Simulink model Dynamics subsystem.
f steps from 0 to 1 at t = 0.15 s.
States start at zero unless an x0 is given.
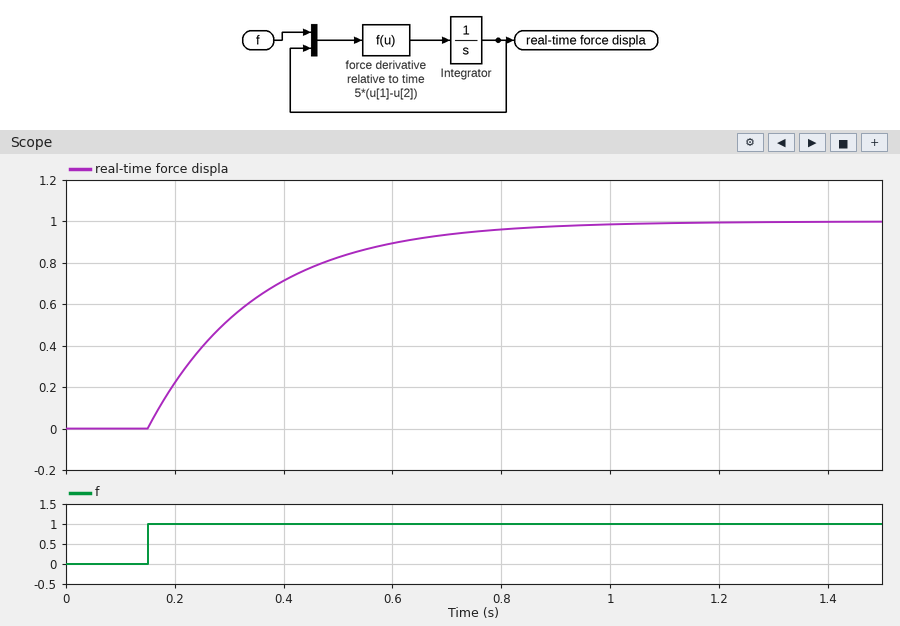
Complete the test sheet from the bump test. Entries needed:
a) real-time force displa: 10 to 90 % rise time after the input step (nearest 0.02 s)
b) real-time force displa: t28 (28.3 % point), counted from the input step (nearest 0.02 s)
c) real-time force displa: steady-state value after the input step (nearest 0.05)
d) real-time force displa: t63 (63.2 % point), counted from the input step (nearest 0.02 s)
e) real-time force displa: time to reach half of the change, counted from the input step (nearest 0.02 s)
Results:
0.44 s
0.06 s
1.00
0.20 s
0.14 s
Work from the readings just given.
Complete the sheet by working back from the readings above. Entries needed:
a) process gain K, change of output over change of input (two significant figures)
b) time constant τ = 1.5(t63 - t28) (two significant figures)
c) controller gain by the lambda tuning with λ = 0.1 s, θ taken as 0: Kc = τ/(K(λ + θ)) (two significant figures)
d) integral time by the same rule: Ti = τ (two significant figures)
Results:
1.0
0.21 s
2.1
0.21 s
